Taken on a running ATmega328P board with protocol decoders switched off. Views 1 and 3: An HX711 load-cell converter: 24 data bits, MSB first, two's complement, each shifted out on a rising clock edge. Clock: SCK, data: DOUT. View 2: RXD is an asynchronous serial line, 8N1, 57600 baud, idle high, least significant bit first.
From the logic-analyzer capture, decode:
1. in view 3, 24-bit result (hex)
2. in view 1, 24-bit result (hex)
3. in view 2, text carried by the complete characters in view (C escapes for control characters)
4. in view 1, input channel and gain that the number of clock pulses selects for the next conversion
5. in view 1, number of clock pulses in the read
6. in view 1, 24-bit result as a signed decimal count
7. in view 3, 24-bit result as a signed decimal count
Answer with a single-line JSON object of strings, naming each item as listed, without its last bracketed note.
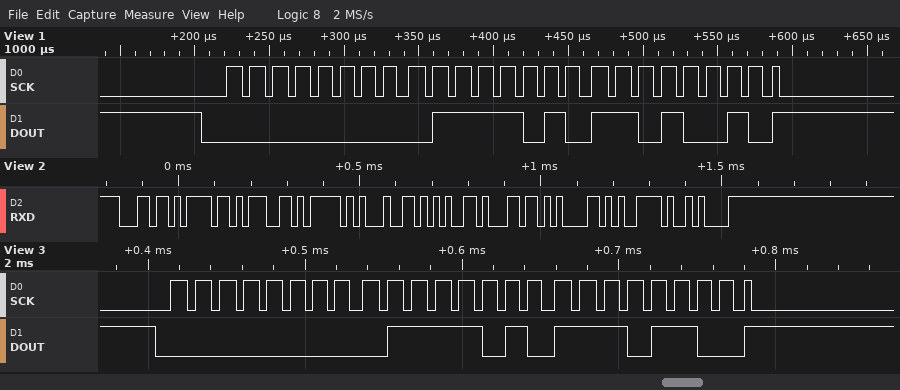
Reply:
{"in view 3, 24-bit result": "0x007AEC", "in view 1, 24-bit result": "0x007AD2", "in view 2, text carried by the complete characters in view": "\"log_delay\\n\"", "in view 1, input channel and gain that the number of clock pulses selects for the next conversion": "channel A, gain 128", "in view 1, number of clock pulses in the read": "25", "in view 1, 24-bit result as a signed decimal count": "31442", "in view 3, 24-bit result as a signed decimal count": "31468"}
